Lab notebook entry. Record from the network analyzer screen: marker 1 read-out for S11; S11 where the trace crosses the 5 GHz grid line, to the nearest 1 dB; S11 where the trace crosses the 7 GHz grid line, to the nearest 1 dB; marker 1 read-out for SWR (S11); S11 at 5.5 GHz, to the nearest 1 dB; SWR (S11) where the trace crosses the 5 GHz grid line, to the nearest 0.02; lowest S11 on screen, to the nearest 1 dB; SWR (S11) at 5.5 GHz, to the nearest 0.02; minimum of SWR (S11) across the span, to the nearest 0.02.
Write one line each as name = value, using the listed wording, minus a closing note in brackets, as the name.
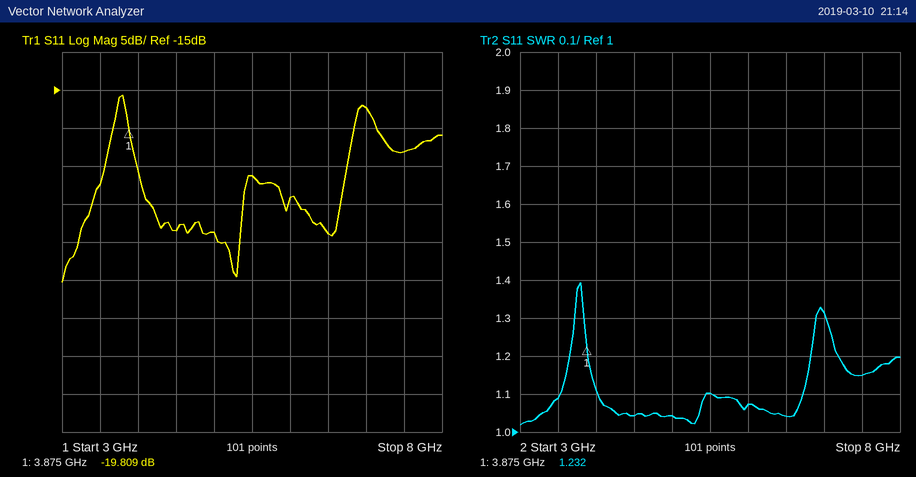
marker 1 read-out for S11 = -19.809 dB
S11 where the trace crosses the 5 GHz grid line, to the nearest 1 dB = -34 dB
S11 where the trace crosses the 7 GHz grid line, to the nearest 1 dB = -17 dB
marker 1 read-out for SWR = 1.232
S11 at 5.5 GHz, to the nearest 1 dB = -26 dB
SWR (S11) where the trace crosses the 5 GHz grid line, to the nearest 0.02 = 1.04
lowest S11 on screen, to the nearest 1 dB = -40 dB
SWR (S11) at 5.5 GHz, to the nearest 0.02 = 1.10
minimum of SWR (S11) across the span, to the nearest 0.02 = 1.02
